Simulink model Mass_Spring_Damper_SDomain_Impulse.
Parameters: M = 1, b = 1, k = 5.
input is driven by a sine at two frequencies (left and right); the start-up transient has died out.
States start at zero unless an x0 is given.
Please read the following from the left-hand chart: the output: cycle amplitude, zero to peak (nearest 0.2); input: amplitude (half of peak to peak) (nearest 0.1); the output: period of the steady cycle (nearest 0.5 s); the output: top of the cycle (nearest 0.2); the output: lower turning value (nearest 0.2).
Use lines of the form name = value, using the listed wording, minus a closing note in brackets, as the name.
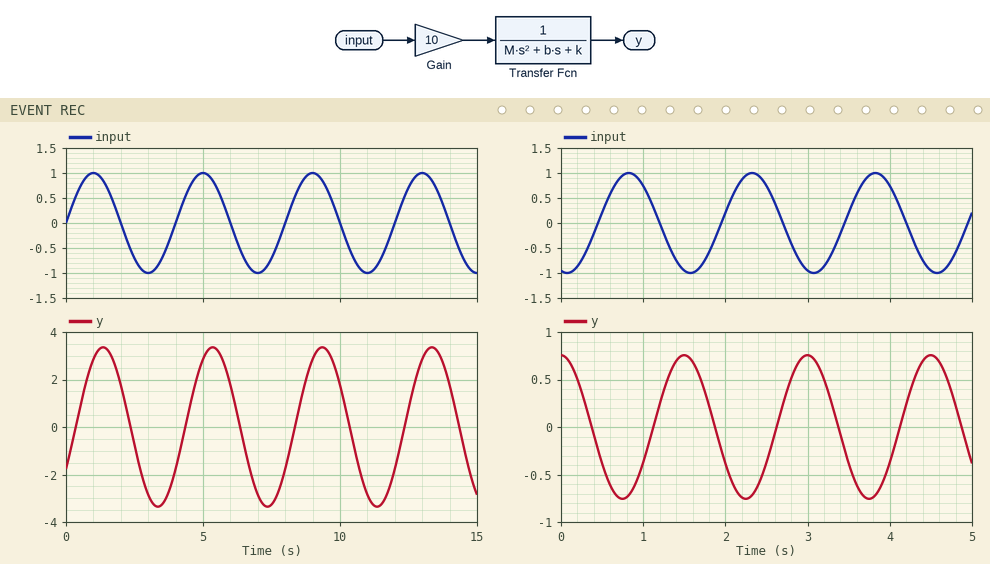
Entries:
the output: cycle amplitude, zero to peak = 3.4
input: amplitude (half of peak to peak) = 1.0
the output: period of the steady cycle = 4.0 s
the output: top of the cycle = 3.4
the output: lower turning value = -3.4
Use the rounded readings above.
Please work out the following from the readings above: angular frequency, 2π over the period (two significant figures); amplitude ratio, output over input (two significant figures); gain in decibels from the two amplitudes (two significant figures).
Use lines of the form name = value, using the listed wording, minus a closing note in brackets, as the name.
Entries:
angular frequency, 2π over the period = 1.6 rad/s
amplitude ratio, output over input = 3.4
gain in decibels from the two amplitudes = 11 dB
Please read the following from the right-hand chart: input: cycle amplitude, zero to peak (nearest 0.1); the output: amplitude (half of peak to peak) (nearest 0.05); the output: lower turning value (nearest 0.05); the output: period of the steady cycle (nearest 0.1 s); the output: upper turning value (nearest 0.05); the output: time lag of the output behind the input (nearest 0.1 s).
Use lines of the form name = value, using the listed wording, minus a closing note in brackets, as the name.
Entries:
input: cycle amplitude, zero to peak = 1.0
the output: amplitude (half of peak to peak) = 0.75
the output: lower turning value = -0.75
the output: period of the steady cycle = 1.5 s
the output: upper turning value = 0.75
the output: time lag of the output behind the input = 0.7 s
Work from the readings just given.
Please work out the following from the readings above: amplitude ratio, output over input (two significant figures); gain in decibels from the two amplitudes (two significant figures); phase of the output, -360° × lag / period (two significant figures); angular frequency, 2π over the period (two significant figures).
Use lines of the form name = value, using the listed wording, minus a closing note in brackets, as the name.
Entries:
amplitude ratio, output over input = 0.75
gain in decibels from the two amplitudes = -2.5 dB
phase of the output, -360° × lag / period = -170°
angular frequency, 2π over the period = 4.2 rad/s
